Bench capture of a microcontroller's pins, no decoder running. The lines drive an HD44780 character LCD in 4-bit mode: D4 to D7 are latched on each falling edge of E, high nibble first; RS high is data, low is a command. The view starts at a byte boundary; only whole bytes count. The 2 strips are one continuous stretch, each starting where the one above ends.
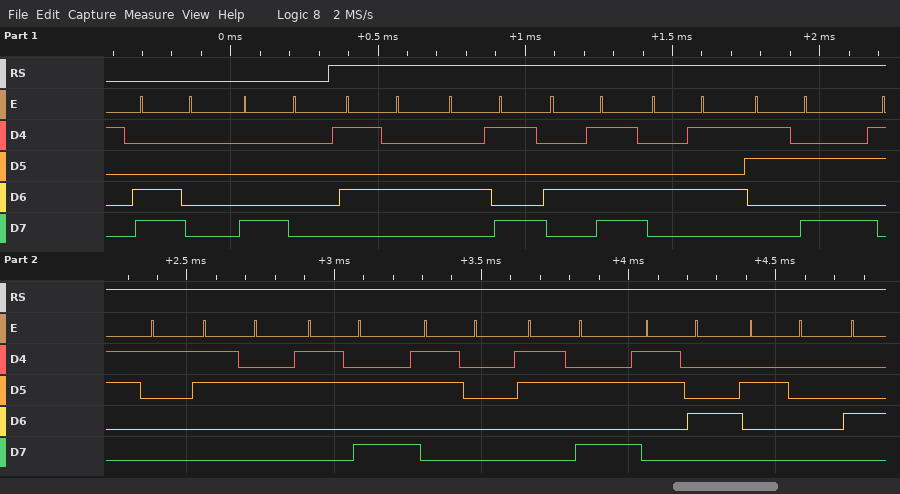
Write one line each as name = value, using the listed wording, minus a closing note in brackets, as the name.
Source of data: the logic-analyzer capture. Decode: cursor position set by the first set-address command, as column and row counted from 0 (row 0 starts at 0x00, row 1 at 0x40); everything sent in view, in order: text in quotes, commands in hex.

cursor position set by the first set-address command, as column and row counted from 0 = column 0, row 1
everything sent in view, in order: text in quotes, commands in hex = 0xC0 0x80 "TIME:12:0:4 "
